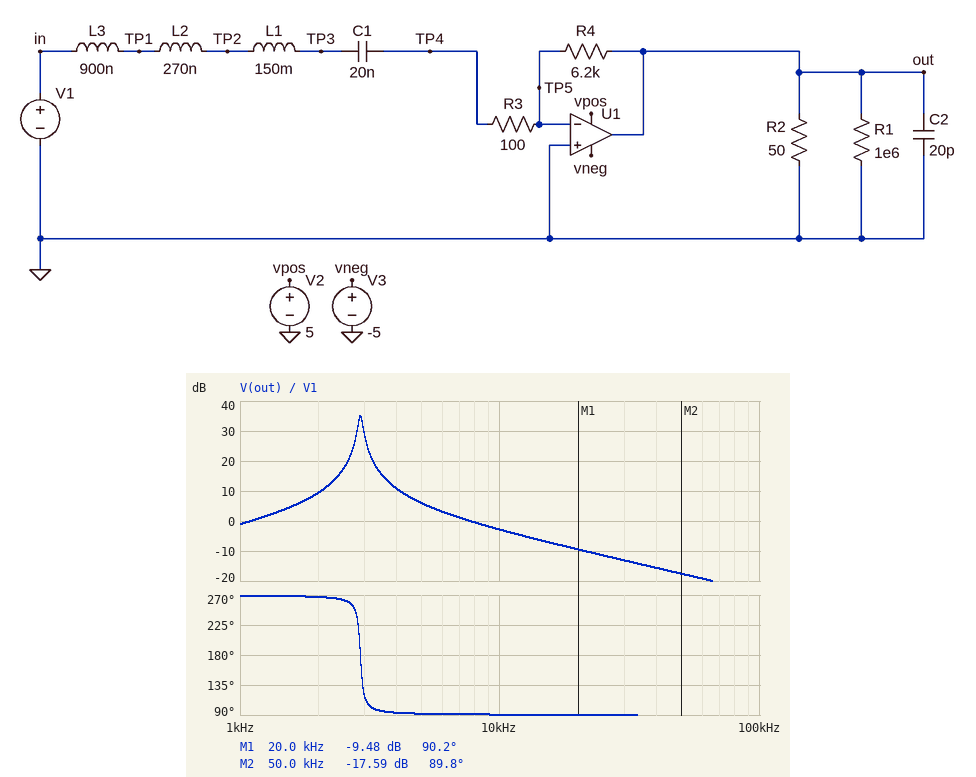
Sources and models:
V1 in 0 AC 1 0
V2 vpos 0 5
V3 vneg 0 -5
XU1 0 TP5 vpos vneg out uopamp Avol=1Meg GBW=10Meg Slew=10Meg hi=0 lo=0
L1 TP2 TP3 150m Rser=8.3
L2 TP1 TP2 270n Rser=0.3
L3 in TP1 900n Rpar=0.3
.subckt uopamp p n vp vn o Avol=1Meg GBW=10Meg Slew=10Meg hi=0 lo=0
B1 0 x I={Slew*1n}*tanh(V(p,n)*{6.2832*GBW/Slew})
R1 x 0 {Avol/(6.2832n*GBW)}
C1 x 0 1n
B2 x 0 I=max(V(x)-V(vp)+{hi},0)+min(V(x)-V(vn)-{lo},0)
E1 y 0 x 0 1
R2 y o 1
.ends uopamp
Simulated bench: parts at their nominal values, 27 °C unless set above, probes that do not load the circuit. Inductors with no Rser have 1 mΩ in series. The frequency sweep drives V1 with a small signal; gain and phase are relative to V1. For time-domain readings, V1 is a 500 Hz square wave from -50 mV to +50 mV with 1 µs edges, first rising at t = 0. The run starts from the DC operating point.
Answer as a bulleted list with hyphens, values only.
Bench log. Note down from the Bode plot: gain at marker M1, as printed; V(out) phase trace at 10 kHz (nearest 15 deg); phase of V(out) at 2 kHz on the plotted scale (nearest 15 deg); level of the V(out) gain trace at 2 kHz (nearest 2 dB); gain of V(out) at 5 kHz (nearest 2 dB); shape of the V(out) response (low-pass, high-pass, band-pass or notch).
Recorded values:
- -9.48 dB
- 90 deg
- 270 deg
- 10 dB
- 6 dB
- band-pass
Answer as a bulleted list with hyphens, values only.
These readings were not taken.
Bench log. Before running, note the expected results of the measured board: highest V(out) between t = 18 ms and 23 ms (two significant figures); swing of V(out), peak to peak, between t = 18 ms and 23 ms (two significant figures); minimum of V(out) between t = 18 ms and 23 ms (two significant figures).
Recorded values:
- 140 mV
- 270 mV
- -140 mV
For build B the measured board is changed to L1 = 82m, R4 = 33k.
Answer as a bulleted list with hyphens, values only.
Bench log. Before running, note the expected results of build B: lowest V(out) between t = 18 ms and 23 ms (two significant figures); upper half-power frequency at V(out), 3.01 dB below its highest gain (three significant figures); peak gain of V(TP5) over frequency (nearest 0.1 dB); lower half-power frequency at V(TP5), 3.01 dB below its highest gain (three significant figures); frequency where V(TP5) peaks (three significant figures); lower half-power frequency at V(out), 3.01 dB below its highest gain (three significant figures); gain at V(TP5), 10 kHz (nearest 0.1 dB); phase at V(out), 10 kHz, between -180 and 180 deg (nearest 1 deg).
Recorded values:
- -1.1 V
- 4.02 kHz
- -18.3 dB
- 3.82 kHz
- 3.92 kHz
- 3.81 kHz
- -42.3 dB
- 91 deg
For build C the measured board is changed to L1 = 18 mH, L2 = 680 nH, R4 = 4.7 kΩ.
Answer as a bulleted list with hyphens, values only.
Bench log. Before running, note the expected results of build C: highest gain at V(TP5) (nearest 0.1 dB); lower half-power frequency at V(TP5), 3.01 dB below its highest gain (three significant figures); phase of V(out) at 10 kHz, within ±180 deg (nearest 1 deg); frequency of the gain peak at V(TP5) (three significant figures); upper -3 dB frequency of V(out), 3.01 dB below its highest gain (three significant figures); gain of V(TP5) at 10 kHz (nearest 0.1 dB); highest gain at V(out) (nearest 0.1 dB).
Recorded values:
- -28.6 dB
- 7.95 kHz
- 108 deg
- 8.40 kHz
- 8.86 kHz
- -37.4 dB
- 32.7 dB
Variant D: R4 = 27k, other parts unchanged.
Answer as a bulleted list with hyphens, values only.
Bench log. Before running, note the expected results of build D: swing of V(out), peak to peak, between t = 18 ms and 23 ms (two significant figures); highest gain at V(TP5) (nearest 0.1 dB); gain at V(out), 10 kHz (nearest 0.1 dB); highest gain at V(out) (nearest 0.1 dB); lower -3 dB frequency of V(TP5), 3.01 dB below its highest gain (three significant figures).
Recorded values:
- 1.2 V
- -22.7 dB
- 9.9 dB
- 47.9 dB
- 2.85 kHz
